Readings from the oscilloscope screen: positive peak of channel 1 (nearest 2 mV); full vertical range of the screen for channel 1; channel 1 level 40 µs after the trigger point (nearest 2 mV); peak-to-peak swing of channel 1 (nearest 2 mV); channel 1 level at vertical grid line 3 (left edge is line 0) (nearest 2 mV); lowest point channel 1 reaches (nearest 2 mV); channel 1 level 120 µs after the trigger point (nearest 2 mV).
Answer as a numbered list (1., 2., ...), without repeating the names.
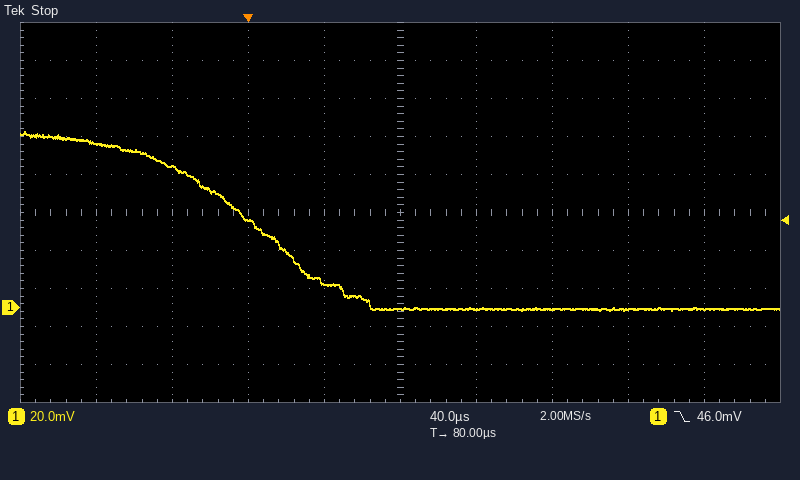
1. 92 mV
2. 200 mV
3. 14 mV
4. 94 mV
5. 46 mV
6. -2 mV
7. 0 mV
